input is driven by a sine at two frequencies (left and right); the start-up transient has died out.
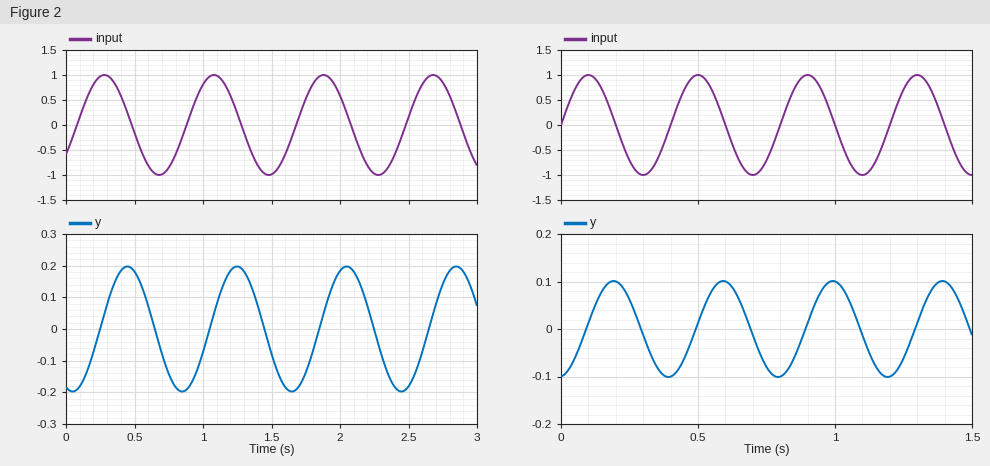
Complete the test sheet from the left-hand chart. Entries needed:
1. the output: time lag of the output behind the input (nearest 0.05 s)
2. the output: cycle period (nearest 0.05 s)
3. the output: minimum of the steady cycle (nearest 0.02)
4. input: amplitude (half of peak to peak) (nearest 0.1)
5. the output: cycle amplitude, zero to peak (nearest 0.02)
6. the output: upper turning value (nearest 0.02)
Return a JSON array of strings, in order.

["0.15 s", "0.80 s", "-0.20", "1.0", "0.20", "0.20"]
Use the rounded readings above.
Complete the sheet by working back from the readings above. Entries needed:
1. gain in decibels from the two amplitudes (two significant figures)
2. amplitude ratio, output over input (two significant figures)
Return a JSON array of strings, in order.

["-14 dB", "0.20"]
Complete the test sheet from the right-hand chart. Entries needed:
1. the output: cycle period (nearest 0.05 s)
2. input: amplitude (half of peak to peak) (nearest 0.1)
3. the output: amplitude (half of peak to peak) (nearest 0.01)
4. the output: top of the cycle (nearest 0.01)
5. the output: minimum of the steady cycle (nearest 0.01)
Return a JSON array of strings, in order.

["0.40 s", "1.0", "0.10", "0.10", "-0.10"]
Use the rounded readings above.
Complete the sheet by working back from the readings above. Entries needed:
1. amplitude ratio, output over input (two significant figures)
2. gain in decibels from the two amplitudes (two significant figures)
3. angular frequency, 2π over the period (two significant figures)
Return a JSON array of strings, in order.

["0.10", "-20 dB", "16 rad/s"]
